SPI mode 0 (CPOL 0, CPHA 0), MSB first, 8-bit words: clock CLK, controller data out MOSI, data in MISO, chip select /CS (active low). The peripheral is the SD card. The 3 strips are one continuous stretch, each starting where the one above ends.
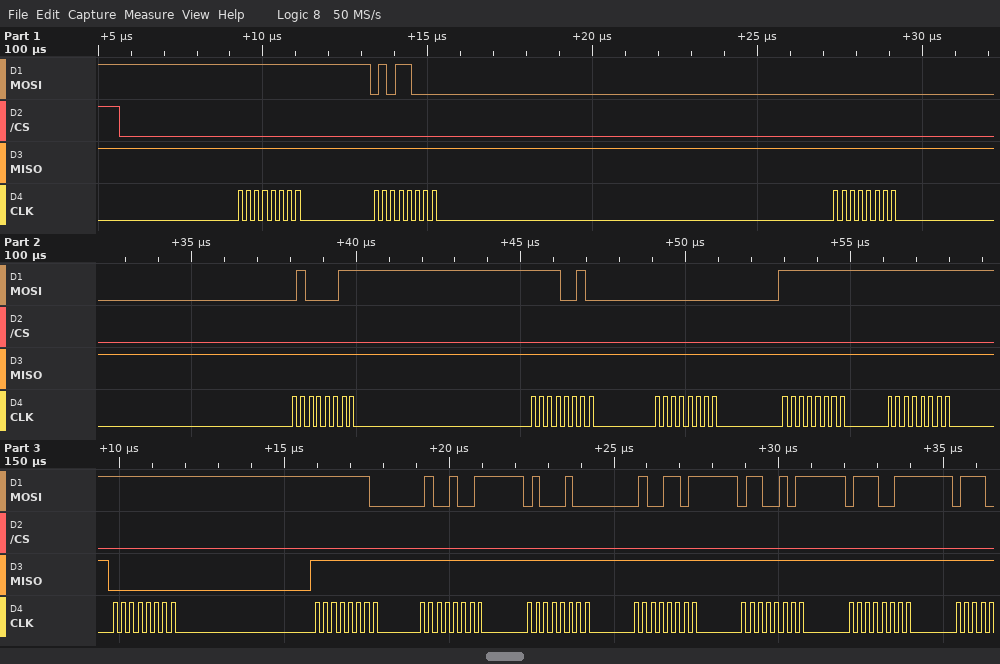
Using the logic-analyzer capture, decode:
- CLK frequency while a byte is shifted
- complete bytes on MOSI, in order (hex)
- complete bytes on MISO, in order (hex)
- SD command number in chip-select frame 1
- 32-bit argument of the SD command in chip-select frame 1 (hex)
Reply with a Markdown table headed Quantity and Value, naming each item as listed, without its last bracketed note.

| Quantity | Value |
|---|---|
| CLK frequency while a byte is shifted | 4 MHz |
| complete bytes on MOSI, in order | FF 58 00 43 F2 00 FF FF FF FE 49 44 4D 65 73 |
| complete bytes on MISO, in order | FF FF FF FF FF FF FF FF 00 FF FF FF FF FF FF |
| SD command number in chip-select frame 1 | CMD24 |
| 32-bit argument of the SD command in chip-select frame 1 | 0x0043F200 |
